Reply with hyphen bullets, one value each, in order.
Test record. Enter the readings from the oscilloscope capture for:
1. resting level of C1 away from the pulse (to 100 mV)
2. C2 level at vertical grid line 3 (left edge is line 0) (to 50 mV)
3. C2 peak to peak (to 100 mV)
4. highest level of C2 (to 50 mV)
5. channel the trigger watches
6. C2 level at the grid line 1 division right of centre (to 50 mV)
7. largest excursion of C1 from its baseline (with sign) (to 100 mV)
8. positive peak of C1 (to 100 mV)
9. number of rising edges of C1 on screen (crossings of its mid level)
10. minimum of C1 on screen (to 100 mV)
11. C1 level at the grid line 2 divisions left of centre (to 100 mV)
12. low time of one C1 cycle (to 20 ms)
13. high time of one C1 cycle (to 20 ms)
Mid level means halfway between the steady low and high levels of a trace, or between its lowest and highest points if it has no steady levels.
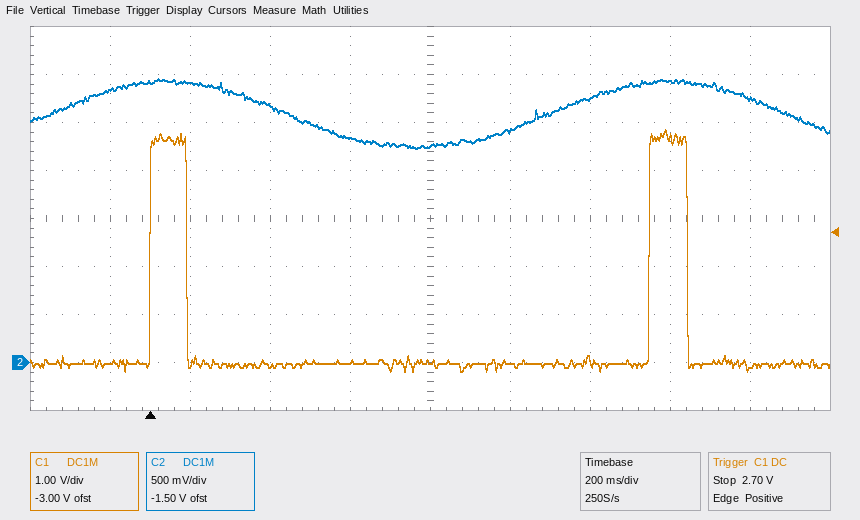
- 0.0 V
- 2.65 V
- 700 mV
- 2.95 V
- C1
- 2.40 V
- +4.9 V
- 4.9 V
- 2
- -200 mV
- -100 mV
- 1.16 s
- 100 ms
